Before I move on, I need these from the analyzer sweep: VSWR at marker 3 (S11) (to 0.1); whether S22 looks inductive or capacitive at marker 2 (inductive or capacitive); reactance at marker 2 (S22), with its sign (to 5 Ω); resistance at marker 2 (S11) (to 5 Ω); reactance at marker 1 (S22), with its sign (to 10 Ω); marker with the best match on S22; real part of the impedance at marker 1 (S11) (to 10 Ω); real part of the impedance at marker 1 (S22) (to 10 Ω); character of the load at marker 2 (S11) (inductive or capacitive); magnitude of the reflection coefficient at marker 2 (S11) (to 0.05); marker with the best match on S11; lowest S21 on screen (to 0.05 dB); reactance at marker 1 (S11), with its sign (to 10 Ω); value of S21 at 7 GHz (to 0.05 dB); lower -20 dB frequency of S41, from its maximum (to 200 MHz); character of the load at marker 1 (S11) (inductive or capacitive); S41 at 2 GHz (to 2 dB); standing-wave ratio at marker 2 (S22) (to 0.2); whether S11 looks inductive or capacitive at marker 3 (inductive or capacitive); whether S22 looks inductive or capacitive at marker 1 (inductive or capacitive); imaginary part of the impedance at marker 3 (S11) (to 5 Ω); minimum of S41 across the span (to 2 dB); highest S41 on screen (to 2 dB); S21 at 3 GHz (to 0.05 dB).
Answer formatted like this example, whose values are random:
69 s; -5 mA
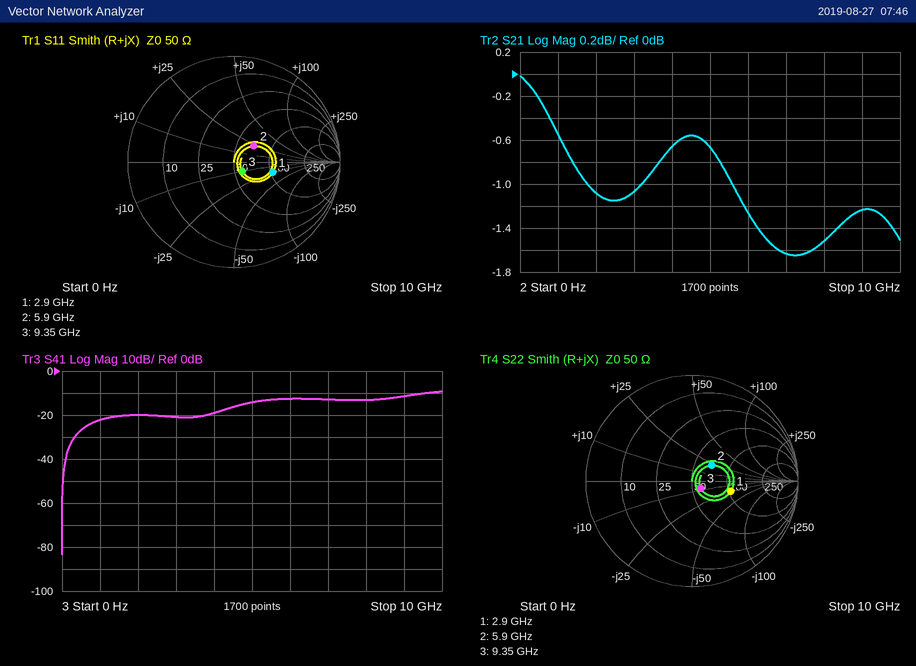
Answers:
1.3; inductive; +20 Ω; 70 Ω; -20 Ω; marker 3; 100 Ω; 100 Ω; inductive; 0.25; marker 3; -1.65 dB; -20 Ω; -1.65 dB; 400 MHz; capacitive; -20 dB; 1.6; capacitive; capacitive; -10 Ω; -84 dB; -10 dB; -1.05 dB
